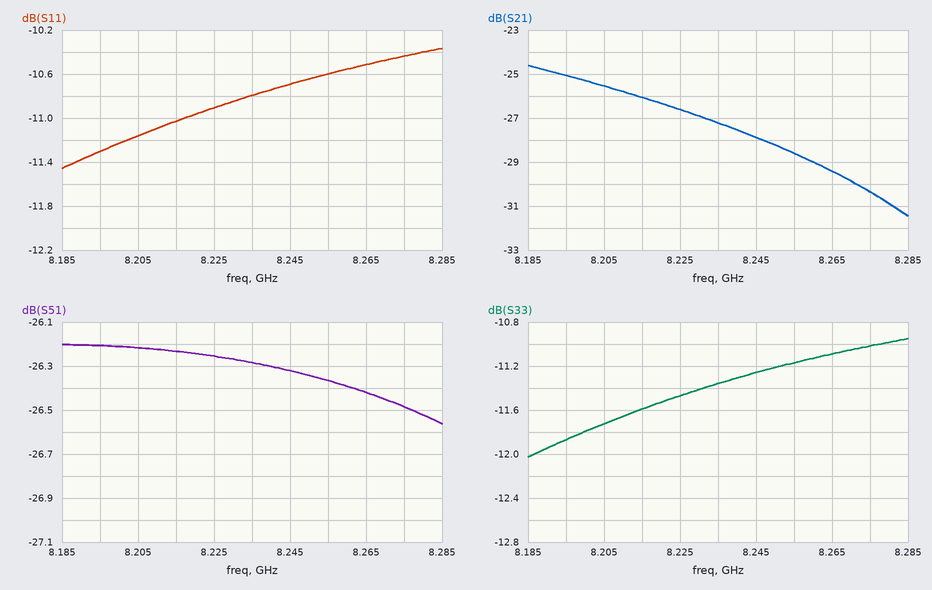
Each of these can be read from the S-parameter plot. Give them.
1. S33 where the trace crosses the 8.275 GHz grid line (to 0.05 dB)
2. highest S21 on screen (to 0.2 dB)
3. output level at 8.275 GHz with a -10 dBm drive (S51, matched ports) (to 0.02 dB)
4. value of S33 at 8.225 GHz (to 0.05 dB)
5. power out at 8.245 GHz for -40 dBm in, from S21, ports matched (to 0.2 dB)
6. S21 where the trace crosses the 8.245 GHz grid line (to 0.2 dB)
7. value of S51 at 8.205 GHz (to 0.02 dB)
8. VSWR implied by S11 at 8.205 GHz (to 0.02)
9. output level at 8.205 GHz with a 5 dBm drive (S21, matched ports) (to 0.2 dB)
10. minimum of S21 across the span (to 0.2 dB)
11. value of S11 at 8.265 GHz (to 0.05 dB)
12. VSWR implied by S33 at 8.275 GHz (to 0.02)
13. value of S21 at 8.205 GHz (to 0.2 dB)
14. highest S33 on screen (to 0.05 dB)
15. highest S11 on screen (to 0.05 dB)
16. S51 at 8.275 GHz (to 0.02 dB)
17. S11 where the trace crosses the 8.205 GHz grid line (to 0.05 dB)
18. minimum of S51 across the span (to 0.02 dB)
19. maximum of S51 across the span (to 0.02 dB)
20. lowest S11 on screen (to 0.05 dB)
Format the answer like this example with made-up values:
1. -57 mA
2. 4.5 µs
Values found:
1. -11.00 dB
2. -24.6 dB
3. -36.48 dBm
4. -11.45 dB
5. -67.8 dBm
6. -27.8 dB
7. -26.22 dB
8. 1.76
9. -20.6 dBm
10. -31.4 dB
11. -10.50 dB
12. 1.78
13. -25.6 dB
14. -10.95 dB
15. -10.35 dB
16. -26.48 dB
17. -11.15 dB
18. -26.56 dB
19. -26.20 dB
20. -11.45 dB
